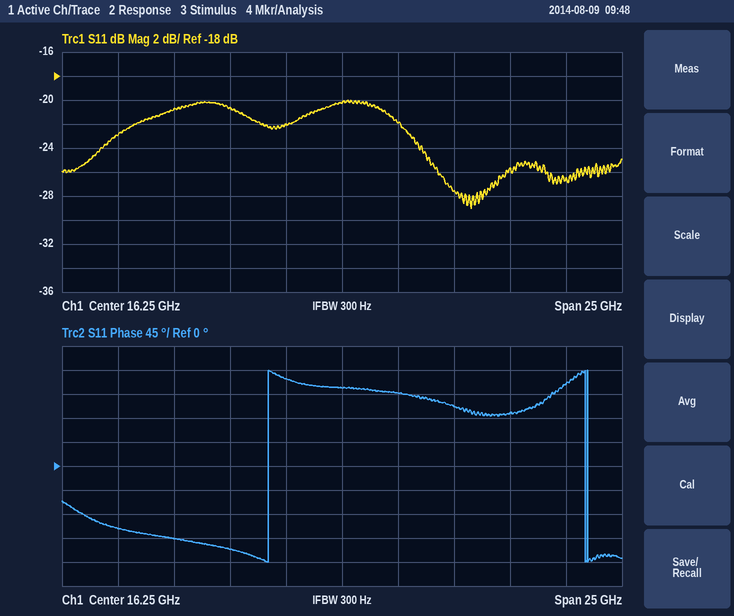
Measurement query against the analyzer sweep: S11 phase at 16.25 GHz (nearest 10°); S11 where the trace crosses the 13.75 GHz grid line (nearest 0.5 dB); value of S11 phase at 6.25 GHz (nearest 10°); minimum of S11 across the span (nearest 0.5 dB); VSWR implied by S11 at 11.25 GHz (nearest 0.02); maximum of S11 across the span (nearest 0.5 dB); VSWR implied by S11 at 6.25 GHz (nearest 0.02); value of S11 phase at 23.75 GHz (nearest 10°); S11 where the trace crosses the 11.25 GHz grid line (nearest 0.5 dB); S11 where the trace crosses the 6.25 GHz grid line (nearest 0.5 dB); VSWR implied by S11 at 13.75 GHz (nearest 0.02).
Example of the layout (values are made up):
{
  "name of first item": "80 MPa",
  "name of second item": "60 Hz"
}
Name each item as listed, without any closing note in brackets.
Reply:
{
  "S11 phase at 16.25 GHz": "150°",
  "S11 where the trace crosses the 13.75 GHz grid line": "-22.0 dB",
  "value of S11 phase at 6.25 GHz": "-120°",
  "minimum of S11 across the span": "-29.0 dB",
  "VSWR implied by S11 at 11.25 GHz": "1.20",
  "maximum of S11 across the span": "-20.0 dB",
  "VSWR implied by S11 at 6.25 GHz": "1.16",
  "value of S11 phase at 23.75 GHz": "100°",
  "S11 where the trace crosses the 11.25 GHz grid line": "-20.5 dB",
  "S11 where the trace crosses the 6.25 GHz grid line": "-23.0 dB",
  "VSWR implied by S11 at 13.75 GHz": "1.18"
}
